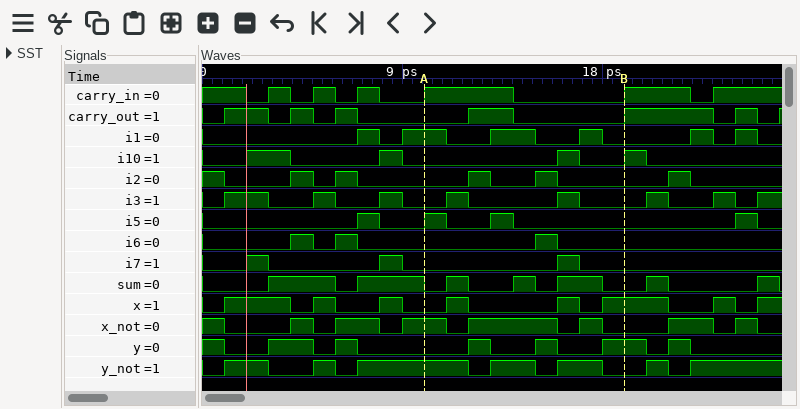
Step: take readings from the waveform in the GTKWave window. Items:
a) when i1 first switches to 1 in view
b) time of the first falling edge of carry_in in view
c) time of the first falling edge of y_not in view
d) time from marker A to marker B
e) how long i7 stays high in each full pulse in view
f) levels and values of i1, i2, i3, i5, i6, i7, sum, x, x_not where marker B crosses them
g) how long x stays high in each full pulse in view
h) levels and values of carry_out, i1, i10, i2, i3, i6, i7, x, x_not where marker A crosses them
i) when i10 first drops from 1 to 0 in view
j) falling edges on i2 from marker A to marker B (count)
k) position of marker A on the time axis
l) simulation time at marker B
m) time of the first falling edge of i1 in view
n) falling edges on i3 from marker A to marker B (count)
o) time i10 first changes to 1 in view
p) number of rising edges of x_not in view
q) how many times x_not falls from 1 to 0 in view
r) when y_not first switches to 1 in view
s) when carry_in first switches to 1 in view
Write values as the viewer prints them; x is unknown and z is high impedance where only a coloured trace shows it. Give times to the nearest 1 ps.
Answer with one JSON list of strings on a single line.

["7 ps", "2 ps", "3 ps", "9 ps", "1 ps, 1 ps, 1 ps", "i1=0, i2=0, i3=0, i5=0, i6=0, i7=0, sum=0, x=1, x_not=0", "3 ps, 1 ps, 1 ps, 1 ps, 1 ps, 3 ps, 1 ps", "carry_out=0, i1=1, i10=0, i2=0, i3=0, i6=0, i7=0, x=0, x_not=1", "4 ps", "2", "10 ps", "19 ps", "8 ps", "2", "2 ps", "7", "8", "1 ps", "3 ps"]
